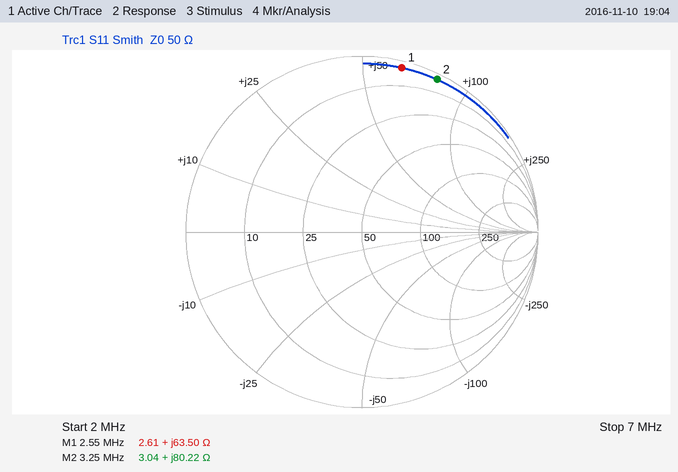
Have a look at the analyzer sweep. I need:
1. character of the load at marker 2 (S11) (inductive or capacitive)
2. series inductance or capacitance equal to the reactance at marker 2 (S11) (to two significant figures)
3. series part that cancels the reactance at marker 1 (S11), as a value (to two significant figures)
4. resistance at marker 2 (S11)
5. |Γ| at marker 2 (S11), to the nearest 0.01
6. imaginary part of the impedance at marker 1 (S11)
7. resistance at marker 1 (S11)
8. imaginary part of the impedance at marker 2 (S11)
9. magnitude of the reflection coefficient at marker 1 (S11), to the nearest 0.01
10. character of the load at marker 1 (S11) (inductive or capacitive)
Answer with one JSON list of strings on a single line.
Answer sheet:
["inductive", "3.9 µH", "980 pF", "3.04 Ω", "0.97", "+63.50 Ω", "2.61 Ω", "+80.22 Ω", "0.96", "inductive"]
